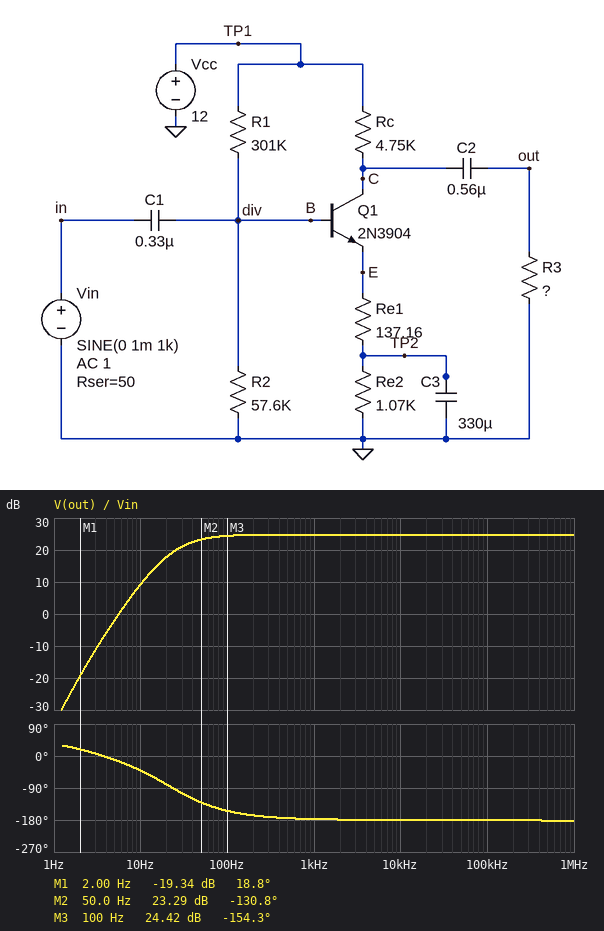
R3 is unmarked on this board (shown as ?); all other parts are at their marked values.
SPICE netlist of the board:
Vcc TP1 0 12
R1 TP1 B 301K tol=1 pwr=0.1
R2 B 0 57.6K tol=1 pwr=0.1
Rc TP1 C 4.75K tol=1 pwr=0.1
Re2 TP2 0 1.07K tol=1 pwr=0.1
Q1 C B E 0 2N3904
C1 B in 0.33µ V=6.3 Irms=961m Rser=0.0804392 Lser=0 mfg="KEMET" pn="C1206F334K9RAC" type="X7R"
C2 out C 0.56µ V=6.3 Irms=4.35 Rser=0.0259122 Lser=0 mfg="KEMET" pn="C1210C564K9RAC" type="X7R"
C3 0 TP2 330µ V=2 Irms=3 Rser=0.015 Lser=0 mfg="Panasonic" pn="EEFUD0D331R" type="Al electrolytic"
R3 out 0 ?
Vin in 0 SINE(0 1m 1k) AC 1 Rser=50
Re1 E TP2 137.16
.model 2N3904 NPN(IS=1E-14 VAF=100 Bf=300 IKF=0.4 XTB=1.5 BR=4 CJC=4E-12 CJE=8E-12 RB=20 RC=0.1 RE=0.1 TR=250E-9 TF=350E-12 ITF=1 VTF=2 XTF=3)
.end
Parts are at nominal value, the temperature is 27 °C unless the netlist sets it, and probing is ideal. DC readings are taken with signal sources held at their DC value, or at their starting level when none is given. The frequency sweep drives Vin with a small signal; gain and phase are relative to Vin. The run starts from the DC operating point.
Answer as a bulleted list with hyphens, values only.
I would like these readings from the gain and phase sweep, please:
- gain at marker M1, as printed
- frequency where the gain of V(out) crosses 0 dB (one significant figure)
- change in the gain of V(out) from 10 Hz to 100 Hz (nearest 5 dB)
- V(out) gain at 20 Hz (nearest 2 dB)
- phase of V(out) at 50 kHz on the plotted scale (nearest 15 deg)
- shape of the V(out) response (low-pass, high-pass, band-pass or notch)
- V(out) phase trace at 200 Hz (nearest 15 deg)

- -19.34 dB
- 6 Hz
- 15 dB
- 18 dB
- -180 deg
- high-pass
- -165 deg
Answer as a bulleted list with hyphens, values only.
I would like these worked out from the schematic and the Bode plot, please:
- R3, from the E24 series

- 7.5 kΩ
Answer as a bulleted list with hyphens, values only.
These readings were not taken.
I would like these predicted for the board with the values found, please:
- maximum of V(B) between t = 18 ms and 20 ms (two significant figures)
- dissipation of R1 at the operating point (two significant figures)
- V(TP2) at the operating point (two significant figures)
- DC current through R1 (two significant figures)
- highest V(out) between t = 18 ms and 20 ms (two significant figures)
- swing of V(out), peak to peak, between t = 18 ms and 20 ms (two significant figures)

- 1.8 V
- 350 µW
- 1.0 V
- 34 µA
- 17 mV
- 35 mV
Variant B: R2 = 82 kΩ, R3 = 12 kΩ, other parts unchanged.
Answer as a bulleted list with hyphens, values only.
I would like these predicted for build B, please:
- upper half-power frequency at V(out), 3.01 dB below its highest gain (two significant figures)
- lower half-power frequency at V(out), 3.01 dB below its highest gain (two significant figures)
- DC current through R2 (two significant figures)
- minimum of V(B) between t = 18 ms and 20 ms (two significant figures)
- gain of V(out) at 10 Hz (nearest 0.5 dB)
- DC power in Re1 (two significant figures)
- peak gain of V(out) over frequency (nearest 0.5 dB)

- 14 MHz
- 29 Hz
- 28 µA
- 2.3 V
- 13.5 dB
- 250 µW
- 26.5 dB
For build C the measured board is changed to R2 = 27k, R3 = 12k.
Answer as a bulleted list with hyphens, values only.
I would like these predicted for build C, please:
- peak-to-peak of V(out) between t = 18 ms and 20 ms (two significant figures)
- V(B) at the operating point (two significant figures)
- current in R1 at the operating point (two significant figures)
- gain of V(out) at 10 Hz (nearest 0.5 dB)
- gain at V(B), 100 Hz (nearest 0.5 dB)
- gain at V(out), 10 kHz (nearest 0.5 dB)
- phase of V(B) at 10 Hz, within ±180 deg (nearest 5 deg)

- 30 mV
- 970 mV
- 37 µA
- 8.5 dB
- -0.5 dB
- 23.5 dB
- 65 deg
